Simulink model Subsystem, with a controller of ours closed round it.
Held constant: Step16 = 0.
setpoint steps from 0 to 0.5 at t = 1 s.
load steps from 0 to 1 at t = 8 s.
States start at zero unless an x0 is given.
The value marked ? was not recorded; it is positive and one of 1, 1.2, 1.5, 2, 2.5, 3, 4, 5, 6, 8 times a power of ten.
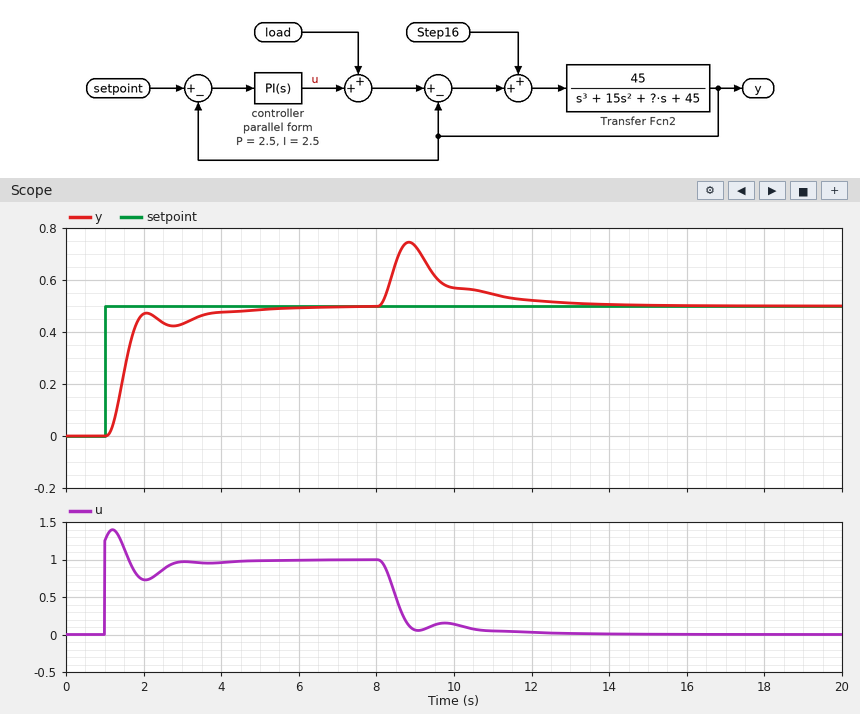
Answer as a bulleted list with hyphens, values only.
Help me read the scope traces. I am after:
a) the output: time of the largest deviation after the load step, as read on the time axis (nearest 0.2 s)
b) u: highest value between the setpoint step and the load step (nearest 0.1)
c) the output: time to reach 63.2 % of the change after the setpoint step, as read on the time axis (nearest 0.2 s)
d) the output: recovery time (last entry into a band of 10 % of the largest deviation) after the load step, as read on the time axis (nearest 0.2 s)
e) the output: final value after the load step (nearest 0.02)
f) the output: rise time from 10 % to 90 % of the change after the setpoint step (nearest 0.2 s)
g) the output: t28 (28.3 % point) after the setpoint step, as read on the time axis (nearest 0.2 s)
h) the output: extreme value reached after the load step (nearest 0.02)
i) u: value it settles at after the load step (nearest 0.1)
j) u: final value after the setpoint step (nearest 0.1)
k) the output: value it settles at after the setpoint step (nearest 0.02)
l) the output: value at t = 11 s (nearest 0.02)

- 8.8 s
- 1.4
- 1.6 s
- 11.8 s
- 0.50
- 0.6 s
- 1.4 s
- 0.74
- 0.0
- 1.0
- 0.50
- 0.54
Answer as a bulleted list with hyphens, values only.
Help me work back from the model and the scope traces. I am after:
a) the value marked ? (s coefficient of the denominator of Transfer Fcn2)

- 60
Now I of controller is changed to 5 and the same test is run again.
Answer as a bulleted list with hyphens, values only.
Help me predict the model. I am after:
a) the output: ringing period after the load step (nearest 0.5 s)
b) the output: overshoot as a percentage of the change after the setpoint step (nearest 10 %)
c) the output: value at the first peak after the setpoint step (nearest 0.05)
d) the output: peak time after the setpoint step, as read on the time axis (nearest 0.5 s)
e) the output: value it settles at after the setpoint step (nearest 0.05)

- 2.0 s
- 20 %
- 0.60
- 2.0 s
- 0.50
